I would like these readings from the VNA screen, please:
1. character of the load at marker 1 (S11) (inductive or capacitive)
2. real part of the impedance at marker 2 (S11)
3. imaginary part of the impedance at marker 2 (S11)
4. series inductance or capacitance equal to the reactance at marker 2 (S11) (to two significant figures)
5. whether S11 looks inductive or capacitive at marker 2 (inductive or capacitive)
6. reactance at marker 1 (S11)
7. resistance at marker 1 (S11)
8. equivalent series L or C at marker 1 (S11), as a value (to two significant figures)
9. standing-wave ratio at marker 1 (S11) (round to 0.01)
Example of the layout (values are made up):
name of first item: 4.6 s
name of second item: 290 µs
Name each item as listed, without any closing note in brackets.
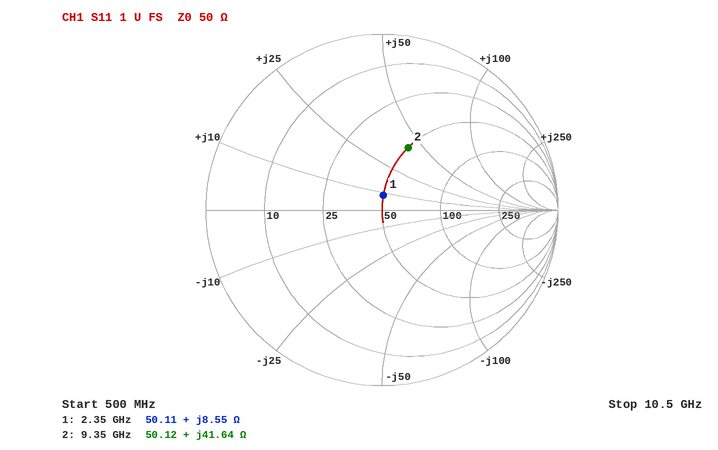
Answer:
character of the load at marker 1 (S11): inductive
real part of the impedance at marker 2: 50.12 Ω
imaginary part of the impedance at marker 2: +41.64 Ω
series inductance or capacitance equal to the reactance at marker 2 (S11): 710 pH
whether S11 looks inductive or capacitive at marker 2: inductive
reactance at marker 1: +8.55 Ω
resistance at marker 1: 50.11 Ω
equivalent series L or C at marker 1 (S11), as a value: 580 pH
standing-wave ratio at marker 1 (S11): 1.19
